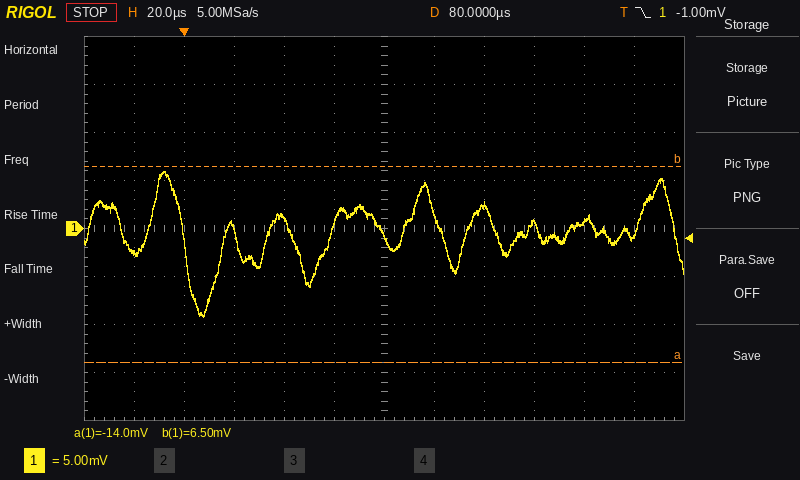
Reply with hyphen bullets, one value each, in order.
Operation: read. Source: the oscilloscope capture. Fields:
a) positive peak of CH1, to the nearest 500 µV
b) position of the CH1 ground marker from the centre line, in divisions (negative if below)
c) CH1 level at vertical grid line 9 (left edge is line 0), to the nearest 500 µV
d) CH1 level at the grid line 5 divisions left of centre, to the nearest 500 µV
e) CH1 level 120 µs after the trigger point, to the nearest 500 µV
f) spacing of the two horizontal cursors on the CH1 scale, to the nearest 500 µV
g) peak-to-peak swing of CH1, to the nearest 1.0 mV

- 6.0 mV
- 0.0 div
- 500 µV
- -2.5 mV
- 2.5 mV
- 20.5 mV
- 15.0 mV
